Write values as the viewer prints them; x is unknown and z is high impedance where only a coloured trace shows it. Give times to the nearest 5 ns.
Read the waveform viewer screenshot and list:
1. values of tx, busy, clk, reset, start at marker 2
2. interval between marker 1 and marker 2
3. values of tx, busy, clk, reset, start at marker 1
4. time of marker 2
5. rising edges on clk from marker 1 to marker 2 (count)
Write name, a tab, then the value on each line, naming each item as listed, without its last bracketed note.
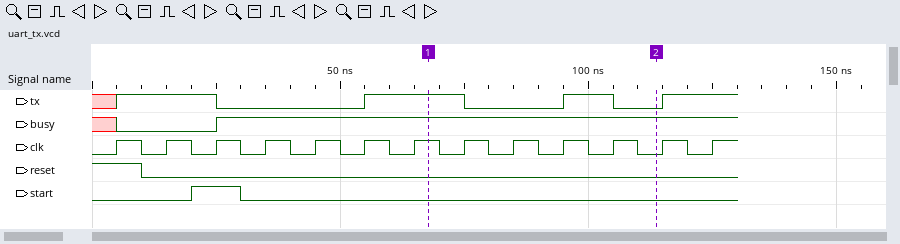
values of tx, busy, clk, reset, start at marker 2	tx=0, busy=1, clk=0, reset=0, start=0
interval between marker 1 and marker 2	45 ns
values of tx, busy, clk, reset, start at marker 1	tx=1, busy=1, clk=1, reset=0, start=0
time of marker 2	115 ns
rising edges on clk from marker 1 to marker 2	4
